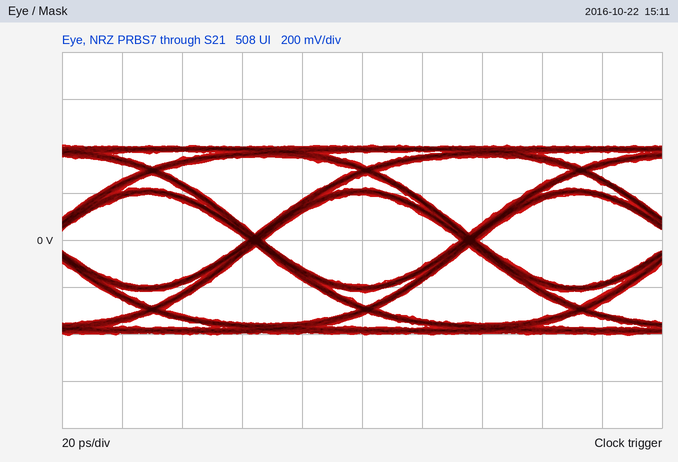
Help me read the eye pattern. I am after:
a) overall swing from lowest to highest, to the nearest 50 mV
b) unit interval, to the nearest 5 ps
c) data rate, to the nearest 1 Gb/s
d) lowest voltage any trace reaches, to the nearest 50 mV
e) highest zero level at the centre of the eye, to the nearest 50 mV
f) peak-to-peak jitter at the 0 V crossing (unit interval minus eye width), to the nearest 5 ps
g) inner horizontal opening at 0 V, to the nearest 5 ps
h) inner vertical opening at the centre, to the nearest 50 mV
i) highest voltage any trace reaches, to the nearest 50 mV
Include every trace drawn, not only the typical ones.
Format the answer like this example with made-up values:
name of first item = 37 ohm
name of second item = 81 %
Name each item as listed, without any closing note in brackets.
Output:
overall swing from lowest to highest, to the nearest 50 mV = 800 mV
unit interval, to the nearest 5 ps = 70 ps
data rate, to the nearest 1 Gb/s = 14 Gb/s
lowest voltage any trace reaches, to the nearest 50 mV = -400 mV
highest zero level at the centre of the eye, to the nearest 50 mV = -200 mV
peak-to-peak jitter at the 0 V crossing (unit interval minus eye width), to the nearest 5 ps = 5 ps
inner horizontal opening at 0 V, to the nearest 5 ps = 65 ps
inner vertical opening at the centre, to the nearest 50 mV = 400 mV
highest voltage any trace reaches, to the nearest 50 mV = 400 mV
